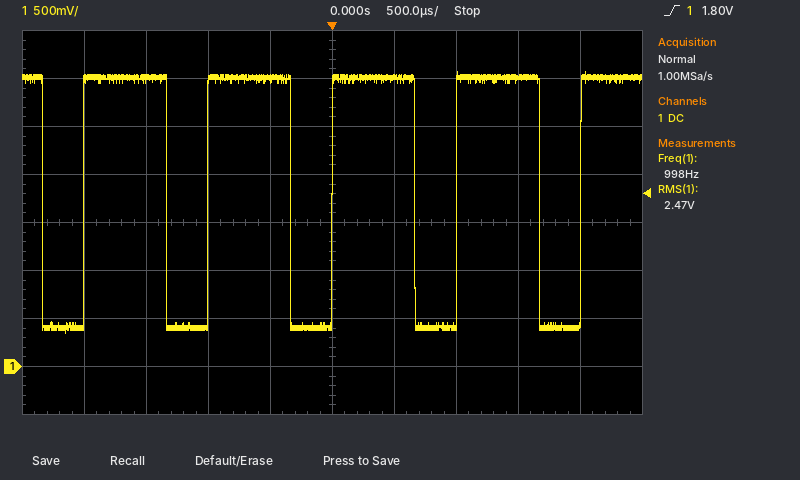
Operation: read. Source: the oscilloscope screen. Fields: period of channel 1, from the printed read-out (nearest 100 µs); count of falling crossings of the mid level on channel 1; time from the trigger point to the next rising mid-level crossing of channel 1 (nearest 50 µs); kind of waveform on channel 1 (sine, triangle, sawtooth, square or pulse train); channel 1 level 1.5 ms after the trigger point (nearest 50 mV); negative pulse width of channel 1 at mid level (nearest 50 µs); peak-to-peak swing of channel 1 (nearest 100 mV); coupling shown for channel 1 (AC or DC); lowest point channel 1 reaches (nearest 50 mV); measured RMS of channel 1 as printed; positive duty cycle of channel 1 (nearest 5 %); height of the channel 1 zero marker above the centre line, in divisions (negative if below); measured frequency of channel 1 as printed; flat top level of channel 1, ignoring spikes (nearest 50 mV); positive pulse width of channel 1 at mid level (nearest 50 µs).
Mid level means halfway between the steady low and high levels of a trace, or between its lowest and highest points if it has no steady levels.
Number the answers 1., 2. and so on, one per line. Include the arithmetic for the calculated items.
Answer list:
1. 1 / 998 Hz ≈ 1.0 ms
2. 5
3. 1.00 ms
4. pulse train
5. 3.00 V
6. 350 µs
7. 2.70 V
8. DC
9. 350 mV
10. 2.47 V
11. 65 %
12. -3.0 div
13. 998 Hz
14. 3.00 V
15. 650 µs
